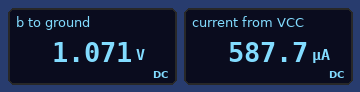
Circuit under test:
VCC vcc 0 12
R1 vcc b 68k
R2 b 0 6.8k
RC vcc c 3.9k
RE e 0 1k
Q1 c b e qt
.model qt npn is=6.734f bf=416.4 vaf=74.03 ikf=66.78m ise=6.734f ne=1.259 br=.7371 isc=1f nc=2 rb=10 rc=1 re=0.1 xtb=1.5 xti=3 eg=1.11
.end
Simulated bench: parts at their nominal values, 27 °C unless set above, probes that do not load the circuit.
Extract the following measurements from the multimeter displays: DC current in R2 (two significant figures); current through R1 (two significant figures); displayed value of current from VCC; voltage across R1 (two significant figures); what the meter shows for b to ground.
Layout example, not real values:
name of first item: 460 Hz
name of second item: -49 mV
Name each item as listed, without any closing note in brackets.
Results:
DC current in R2: 160 µA
current through R1: 160 µA
displayed value of current from VCC: 587.7 µA
voltage across R1: 11 V
what the meter shows for b to ground: 1.071 V
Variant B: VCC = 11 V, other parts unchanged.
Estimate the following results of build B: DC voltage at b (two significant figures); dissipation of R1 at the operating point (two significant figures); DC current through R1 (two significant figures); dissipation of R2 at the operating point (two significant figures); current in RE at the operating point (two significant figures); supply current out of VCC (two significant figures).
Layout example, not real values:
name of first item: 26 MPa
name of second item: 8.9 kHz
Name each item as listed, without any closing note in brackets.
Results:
DC voltage at b: 980 mV
dissipation of R1 at the operating point: 1.5 mW
DC current through R1: 150 µA
dissipation of R2 at the operating point: 140 µW
current in RE at the operating point: 350 µA
supply current out of VCC: 490 µA
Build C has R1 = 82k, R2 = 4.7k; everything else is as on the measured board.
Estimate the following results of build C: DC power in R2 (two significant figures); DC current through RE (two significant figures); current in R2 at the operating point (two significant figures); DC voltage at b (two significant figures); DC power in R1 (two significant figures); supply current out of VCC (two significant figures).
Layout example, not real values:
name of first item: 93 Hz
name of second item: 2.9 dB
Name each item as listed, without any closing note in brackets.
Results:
DC power in R2: 89 µW
DC current through RE: 59 µA
current in R2 at the operating point: 140 µA
DC voltage at b: 650 mV
DC power in R1: 1.6 mW
supply current out of VCC: 200 µA
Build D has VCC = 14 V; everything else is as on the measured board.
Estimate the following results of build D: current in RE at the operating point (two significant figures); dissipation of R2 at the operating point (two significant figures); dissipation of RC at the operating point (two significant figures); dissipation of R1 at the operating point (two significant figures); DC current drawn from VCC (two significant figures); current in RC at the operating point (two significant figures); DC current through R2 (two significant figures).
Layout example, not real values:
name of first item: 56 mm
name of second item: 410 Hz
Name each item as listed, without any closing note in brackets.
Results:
current in RE at the operating point: 600 µA
dissipation of R2 at the operating point: 230 µW
dissipation of RC at the operating point: 1.4 mW
dissipation of R1 at the operating point: 2.4 mW
DC current drawn from VCC: 780 µA
current in RC at the operating point: 590 µA
DC current through R2: 180 µA
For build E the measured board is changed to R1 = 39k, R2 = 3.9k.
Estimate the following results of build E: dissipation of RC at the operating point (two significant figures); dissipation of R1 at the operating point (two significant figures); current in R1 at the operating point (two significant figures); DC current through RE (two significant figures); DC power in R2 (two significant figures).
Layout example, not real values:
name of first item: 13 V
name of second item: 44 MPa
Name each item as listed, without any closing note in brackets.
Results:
dissipation of RC at the operating point: 740 µW
dissipation of R1 at the operating point: 3.1 mW
current in R1 at the operating point: 280 µA
DC current through RE: 440 µA
DC power in R2: 300 µW
